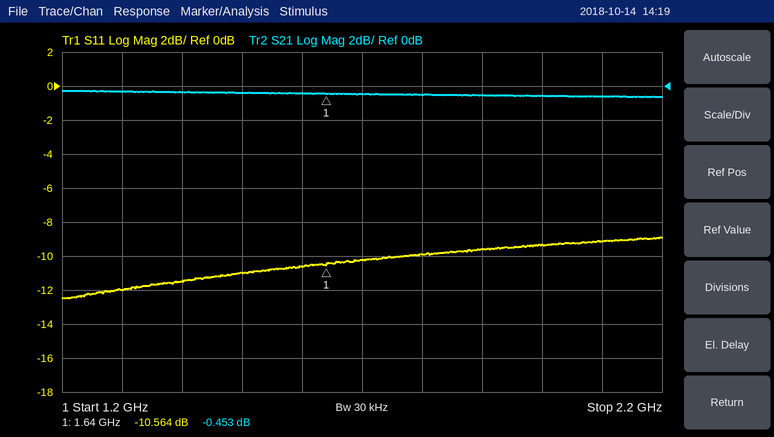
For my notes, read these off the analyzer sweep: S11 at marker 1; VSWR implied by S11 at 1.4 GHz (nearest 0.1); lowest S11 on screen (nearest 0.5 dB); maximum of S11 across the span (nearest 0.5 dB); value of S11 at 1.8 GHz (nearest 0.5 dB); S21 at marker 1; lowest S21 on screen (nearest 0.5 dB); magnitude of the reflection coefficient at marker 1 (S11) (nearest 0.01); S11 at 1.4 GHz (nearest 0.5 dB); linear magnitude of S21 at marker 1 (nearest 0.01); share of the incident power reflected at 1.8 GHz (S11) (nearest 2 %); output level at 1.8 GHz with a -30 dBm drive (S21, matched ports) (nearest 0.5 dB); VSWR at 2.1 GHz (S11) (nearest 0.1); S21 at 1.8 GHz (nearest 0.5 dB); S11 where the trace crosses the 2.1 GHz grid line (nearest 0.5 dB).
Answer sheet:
-10.564 dB
1.7
-12.5 dB
-9.0 dB
-10.0 dB
-0.453 dB
-0.5 dB
0.30
-11.5 dB
0.95
10 %
-30.5 dBm
2.1
-0.5 dB
-9.0 dB
